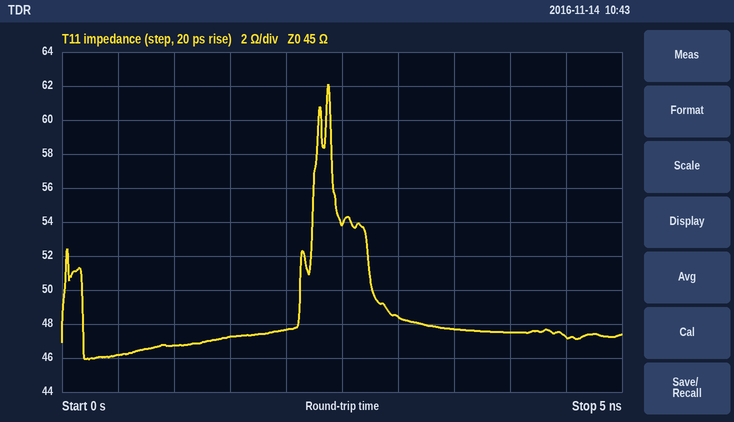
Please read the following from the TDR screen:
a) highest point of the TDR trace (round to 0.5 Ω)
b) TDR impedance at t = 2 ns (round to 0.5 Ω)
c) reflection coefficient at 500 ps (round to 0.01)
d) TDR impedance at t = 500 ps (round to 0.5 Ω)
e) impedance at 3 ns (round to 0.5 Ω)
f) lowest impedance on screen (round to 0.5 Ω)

62.0 Ω
47.5 Ω
+0.01
46.0 Ω
48.5 Ω
46.0 Ω
